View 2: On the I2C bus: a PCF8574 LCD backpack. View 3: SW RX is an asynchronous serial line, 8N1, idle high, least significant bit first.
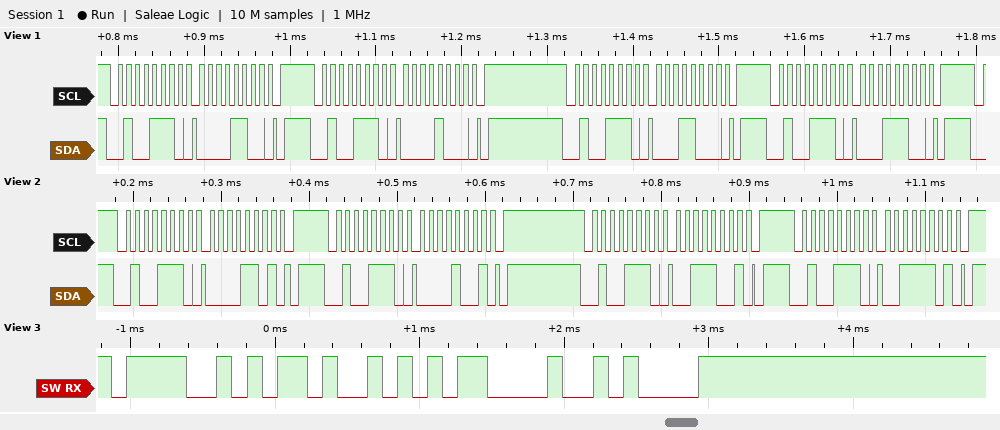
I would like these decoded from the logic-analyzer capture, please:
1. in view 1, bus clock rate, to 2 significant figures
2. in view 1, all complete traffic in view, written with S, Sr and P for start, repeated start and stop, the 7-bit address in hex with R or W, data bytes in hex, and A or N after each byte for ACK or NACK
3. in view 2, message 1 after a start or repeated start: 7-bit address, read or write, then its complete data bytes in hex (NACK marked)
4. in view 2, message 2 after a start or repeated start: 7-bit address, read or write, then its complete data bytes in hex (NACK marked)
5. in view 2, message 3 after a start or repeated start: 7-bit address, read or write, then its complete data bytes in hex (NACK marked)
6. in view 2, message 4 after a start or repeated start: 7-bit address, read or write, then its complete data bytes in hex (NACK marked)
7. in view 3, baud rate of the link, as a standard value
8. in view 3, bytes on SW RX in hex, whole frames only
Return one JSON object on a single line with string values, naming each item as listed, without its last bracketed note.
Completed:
{"in view 1, bus clock rate, to 2 significant figures": "100 kHz", "in view 1, all complete traffic in view, written with S, Sr and P for start, repeated start and stop, the 7-bit address in hex with R or W, data bytes in hex, and A or N after each byte for ACK or NACK": "S 27W A 0C A P S 27W A 08 A P S 27W A 18 A P S 27W A 1C A P", "in view 2, message 1 after a start or repeated start: 7-bit address, read or write, then its complete data bytes in hex": "0x27 write: 0D", "in view 2, message 2 after a start or repeated start: 7-bit address, read or write, then its complete data bytes in hex": "0x27 write: 09", "in view 2, message 3 after a start or repeated start: 7-bit address, read or write, then its complete data bytes in hex": "0x27 write: 39", "in view 2, message 4 after a start or repeated start: 7-bit address, read or write, then its complete data bytes in hex": "0x27 write: 3D", "in view 3, baud rate of the link, as a standard value": "9600 baud", "in view 3, bytes on SW RX in hex, whole frames only": "4F 4B 0D 0A"}
